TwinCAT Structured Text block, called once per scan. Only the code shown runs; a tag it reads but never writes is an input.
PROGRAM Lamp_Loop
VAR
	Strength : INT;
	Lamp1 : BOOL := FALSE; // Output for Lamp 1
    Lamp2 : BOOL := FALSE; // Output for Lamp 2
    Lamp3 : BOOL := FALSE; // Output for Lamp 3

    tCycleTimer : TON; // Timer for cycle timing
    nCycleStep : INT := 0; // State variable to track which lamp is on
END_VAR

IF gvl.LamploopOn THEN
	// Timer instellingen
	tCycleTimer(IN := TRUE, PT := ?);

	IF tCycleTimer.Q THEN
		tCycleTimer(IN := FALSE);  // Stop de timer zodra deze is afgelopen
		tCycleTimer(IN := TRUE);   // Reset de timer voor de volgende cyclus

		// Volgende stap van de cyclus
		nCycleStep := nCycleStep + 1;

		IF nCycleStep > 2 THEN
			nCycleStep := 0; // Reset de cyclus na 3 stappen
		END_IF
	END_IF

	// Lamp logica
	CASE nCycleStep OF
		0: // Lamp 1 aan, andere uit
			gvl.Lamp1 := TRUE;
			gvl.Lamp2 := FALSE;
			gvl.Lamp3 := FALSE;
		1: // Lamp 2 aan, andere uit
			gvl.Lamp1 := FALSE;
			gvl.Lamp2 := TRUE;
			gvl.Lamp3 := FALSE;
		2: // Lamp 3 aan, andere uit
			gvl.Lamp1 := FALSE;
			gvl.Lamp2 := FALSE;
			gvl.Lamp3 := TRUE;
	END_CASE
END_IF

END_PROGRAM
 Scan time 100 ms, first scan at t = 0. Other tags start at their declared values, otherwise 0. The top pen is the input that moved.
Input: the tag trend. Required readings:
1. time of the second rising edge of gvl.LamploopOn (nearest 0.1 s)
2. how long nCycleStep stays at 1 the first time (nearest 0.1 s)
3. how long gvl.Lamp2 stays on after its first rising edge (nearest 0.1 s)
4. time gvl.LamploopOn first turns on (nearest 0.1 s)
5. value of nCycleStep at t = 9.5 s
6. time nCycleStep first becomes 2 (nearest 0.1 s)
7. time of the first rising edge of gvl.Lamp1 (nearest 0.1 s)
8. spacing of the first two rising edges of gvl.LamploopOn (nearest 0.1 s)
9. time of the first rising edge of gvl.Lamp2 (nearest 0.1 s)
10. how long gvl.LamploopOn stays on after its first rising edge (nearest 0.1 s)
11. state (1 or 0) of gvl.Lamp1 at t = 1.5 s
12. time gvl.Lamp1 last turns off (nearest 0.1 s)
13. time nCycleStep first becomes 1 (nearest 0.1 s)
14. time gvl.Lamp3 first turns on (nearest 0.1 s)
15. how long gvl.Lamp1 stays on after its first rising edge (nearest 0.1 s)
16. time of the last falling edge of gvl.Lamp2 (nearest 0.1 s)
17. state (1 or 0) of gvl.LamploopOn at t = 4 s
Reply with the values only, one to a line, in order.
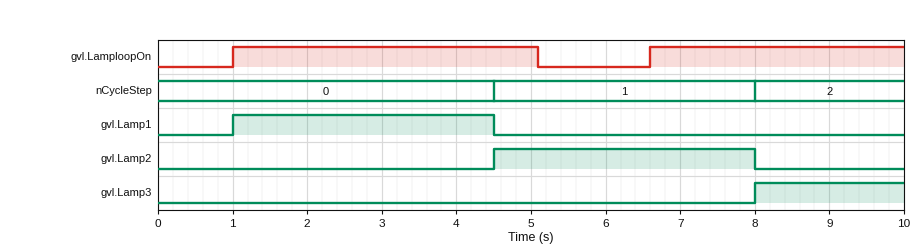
6.6 s
3.5 s
3.5 s
1.0 s
2
8.0 s
1.0 s
5.6 s
4.5 s
4.1 s
1
4.5 s
4.5 s
8.0 s
3.5 s
8.0 s
1
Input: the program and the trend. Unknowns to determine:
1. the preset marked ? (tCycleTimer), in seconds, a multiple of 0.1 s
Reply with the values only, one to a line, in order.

3.5 s
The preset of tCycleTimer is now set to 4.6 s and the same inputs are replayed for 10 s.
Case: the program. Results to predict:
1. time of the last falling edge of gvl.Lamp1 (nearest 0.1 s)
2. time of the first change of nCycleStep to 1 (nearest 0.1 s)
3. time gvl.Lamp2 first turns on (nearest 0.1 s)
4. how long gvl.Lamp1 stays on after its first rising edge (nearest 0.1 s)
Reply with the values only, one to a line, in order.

6.6 s
6.6 s
6.6 s
5.6 s
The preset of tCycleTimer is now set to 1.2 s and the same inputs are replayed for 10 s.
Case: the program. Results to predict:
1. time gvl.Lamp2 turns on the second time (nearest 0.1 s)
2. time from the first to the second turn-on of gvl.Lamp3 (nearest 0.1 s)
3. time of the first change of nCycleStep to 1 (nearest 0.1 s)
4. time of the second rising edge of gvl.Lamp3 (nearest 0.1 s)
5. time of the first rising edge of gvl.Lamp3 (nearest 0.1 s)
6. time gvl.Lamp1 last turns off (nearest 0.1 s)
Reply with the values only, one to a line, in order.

6.6 s
4.4 s
2.2 s
7.8 s
3.4 s
6.6 s
